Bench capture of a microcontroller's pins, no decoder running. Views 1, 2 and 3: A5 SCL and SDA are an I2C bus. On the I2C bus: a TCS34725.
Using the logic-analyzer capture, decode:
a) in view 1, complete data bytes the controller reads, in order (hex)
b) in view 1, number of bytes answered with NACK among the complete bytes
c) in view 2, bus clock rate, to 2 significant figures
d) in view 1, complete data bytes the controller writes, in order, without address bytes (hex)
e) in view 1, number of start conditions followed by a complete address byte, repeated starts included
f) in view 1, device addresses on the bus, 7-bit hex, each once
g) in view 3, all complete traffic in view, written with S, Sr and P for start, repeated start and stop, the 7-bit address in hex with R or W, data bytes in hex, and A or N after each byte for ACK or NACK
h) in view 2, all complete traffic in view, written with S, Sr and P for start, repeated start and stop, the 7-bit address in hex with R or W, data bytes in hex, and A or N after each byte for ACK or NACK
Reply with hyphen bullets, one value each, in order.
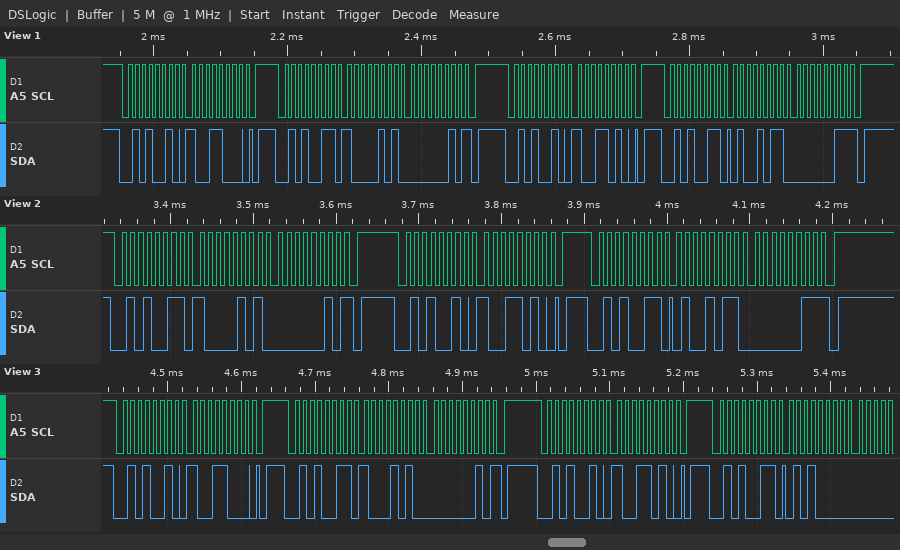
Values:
- 85 02 4B 03
- 2
- 100 kHz
- 98 9A
- 4
- 0x29
- S 29W A 98 A P S 29R A 8A A 02 N P S 29W A 9A A P S 29R A 50 A
- S 29R A 85 A 02 N P S 29W A 9A A P S 29R A 4B A 03 N P
